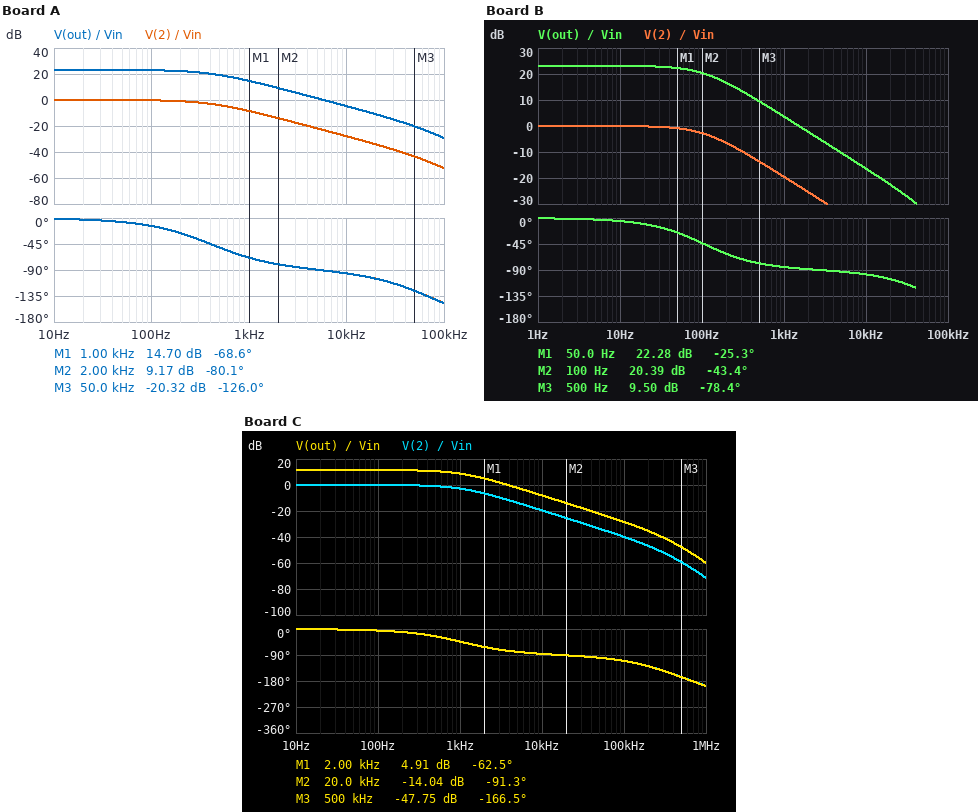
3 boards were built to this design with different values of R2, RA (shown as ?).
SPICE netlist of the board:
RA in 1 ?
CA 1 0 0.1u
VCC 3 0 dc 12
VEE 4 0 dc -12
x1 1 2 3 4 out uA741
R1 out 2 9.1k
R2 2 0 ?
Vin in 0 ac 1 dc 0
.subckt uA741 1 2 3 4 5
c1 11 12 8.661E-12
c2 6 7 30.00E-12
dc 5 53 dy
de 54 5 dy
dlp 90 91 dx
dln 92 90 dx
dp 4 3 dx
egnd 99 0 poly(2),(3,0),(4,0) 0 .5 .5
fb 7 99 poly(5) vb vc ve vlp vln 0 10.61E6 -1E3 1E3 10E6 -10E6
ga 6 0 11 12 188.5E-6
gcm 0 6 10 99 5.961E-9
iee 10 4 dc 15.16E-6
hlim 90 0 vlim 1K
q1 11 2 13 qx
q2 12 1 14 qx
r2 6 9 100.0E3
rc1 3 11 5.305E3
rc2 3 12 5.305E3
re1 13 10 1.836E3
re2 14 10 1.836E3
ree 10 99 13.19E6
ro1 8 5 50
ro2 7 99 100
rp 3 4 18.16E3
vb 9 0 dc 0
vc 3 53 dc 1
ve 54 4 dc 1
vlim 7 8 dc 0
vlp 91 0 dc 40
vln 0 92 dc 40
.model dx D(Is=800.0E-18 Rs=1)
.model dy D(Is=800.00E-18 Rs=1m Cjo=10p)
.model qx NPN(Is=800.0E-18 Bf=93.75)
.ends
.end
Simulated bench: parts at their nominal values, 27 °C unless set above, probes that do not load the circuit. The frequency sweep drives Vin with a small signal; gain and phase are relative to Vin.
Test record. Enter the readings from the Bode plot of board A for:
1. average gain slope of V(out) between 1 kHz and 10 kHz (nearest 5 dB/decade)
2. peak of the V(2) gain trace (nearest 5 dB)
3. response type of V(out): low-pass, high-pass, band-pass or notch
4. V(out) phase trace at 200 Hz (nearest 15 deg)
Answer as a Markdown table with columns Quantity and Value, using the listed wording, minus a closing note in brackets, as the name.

| Quantity | Value |
|---|---|
| average gain slope of V(out) between 1 kHz and 10 kHz | -20 dB/decade |
| peak of the V(2) gain trace | 0 dB |
| response type of V(out): low-pass, high-pass, band-pass or notch | low-pass |
| V(out) phase trace at 200 Hz | -30 deg |
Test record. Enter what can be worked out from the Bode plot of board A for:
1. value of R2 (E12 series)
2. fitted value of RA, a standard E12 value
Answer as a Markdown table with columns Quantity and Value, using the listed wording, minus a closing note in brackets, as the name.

| Quantity | Value |
|---|---|
| value of R2 | 680 Ω |
| fitted value of RA, a standard E12 value | 3.9 kΩ |
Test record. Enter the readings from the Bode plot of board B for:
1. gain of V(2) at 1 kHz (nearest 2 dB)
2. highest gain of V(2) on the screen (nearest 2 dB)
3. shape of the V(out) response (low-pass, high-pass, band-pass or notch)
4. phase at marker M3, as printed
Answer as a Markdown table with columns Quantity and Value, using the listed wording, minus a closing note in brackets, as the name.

| Quantity | Value |
|---|---|
| gain of V(2) at 1 kHz | -20 dB |
| highest gain of V(2) on the screen | 0 dB |
| shape of the V(out) response | low-pass |
| phase at marker M3, as printed | -78.4 deg |
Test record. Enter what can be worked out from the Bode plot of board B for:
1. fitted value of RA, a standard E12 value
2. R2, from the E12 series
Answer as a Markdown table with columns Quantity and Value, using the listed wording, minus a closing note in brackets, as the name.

| Quantity | Value |
|---|---|
| fitted value of RA, a standard E12 value | 15 kΩ |
| R2, from the E12 series | 680 Ω |
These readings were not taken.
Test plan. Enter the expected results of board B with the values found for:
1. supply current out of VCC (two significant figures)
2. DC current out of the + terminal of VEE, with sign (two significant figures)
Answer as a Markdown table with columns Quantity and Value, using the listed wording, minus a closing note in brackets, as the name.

| Quantity | Value |
|---|---|
| supply current out of VCC | 1.3 mA |
| DC current out of the + terminal of VEE, with sign | -1.3 mA |
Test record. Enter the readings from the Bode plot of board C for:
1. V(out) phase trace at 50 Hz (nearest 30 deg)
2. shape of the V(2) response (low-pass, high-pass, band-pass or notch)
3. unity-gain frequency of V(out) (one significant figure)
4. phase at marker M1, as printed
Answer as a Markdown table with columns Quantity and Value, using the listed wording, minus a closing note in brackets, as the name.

| Quantity | Value |
|---|---|
| V(out) phase trace at 50 Hz | 0 deg |
| shape of the V(2) response | low-pass |
| unity-gain frequency of V(out) | 4 kHz |
| phase at marker M1, as printed | -62.5 deg |
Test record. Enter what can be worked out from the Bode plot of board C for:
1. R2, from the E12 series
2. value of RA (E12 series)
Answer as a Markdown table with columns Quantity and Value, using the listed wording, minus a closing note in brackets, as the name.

| Quantity | Value |
|---|---|
| R2, from the E12 series | 3.3 kΩ |
| value of RA | 1.5 kΩ |
